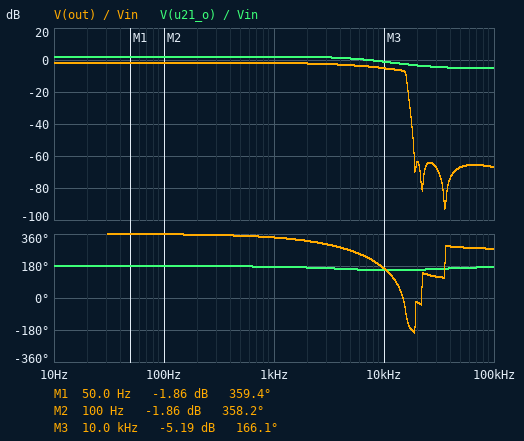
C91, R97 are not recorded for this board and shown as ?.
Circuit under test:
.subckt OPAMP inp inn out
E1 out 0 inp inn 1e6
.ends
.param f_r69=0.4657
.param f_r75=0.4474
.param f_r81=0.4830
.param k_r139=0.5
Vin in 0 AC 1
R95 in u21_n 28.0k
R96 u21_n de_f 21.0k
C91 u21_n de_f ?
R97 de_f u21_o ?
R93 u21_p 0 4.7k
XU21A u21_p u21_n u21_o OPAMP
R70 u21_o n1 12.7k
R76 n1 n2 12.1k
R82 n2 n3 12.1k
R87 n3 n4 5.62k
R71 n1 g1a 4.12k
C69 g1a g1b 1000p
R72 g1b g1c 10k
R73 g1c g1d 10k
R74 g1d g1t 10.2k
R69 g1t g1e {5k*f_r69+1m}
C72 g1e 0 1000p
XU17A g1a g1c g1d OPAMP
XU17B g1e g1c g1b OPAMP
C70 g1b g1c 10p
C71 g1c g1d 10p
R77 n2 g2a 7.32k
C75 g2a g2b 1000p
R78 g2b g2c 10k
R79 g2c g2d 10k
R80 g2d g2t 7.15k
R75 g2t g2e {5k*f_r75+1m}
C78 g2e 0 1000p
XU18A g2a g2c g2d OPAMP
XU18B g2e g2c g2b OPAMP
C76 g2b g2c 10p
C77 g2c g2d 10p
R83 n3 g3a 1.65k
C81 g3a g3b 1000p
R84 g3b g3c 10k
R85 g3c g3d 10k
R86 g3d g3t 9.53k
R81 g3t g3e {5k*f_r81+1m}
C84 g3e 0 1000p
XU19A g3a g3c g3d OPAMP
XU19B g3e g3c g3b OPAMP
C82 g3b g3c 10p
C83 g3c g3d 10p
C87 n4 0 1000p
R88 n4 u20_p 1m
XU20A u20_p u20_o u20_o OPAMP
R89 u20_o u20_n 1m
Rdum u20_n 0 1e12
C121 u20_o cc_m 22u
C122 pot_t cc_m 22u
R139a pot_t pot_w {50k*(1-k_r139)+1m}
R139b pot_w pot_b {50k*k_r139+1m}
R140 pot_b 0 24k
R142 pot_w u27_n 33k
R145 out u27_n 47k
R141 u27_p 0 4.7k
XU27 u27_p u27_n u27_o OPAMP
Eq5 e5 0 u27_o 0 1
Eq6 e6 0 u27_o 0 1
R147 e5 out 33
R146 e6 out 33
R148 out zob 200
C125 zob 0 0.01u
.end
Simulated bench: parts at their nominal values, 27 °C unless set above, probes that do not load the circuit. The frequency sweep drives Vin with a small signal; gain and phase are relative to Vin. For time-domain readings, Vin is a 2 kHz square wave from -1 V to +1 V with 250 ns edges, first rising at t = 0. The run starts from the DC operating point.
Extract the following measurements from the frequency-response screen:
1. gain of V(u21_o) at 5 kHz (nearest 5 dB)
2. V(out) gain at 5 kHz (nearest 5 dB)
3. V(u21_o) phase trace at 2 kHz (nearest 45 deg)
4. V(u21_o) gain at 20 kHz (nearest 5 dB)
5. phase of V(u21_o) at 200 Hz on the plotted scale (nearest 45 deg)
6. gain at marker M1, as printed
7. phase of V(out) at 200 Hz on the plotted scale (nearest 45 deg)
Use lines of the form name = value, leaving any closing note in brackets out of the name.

gain of V(u21_o) at 5 kHz = 0 dB
V(out) gain at 5 kHz = -5 dB
V(u21_o) phase trace at 2 kHz = 180 deg
V(u21_o) gain at 20 kHz = -5 dB
phase of V(u21_o) at 200 Hz on the plotted scale = 180 deg
gain at marker M1, as printed = -1.86 dB
phase of V(out) at 200 Hz on the plotted scale = 360 deg
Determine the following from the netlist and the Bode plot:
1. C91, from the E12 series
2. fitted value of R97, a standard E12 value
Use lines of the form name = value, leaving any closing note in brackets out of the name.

C91, from the E12 series = 1 nF
fitted value of R97, a standard E12 value = 15 kΩ
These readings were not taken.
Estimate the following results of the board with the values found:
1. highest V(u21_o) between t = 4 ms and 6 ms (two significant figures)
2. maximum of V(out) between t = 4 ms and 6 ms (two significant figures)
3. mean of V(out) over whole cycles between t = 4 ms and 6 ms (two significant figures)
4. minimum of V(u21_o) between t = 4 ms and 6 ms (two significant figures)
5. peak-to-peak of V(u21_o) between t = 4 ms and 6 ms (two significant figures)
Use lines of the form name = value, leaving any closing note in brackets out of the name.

highest V(u21_o) between t = 4 ms and 6 ms = 1.3 V
maximum of V(out) between t = 4 ms and 6 ms = 1.7 V
mean of V(out) over whole cycles between t = 4 ms and 6 ms = 800 mV
minimum of V(u21_o) between t = 4 ms and 6 ms = -1.3 V
peak-to-peak of V(u21_o) between t = 4 ms and 6 ms = 2.6 V
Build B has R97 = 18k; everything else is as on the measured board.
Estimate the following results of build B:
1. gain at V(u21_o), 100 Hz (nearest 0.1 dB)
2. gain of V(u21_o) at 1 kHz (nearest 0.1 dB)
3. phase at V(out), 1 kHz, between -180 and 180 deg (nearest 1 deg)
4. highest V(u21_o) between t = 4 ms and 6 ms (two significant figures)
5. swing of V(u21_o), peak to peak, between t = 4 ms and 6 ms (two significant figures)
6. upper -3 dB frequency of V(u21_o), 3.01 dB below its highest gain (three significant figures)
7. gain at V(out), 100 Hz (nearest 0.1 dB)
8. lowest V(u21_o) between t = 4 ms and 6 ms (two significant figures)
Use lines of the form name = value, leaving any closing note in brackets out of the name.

gain at V(u21_o), 100 Hz = 2.9 dB
gain of V(u21_o) at 1 kHz = 2.8 dB
phase at V(out), 1 kHz, between -180 and 180 deg = -19 deg
highest V(u21_o) between t = 4 ms and 6 ms = 1.4 V
swing of V(u21_o), peak to peak, between t = 4 ms and 6 ms = 2.8 V
upper -3 dB frequency of V(u21_o), 3.01 dB below its highest gain = 10.0 kHz
gain at V(out), 100 Hz = -1.2 dB
lowest V(u21_o) between t = 4 ms and 6 ms = -1.4 V
